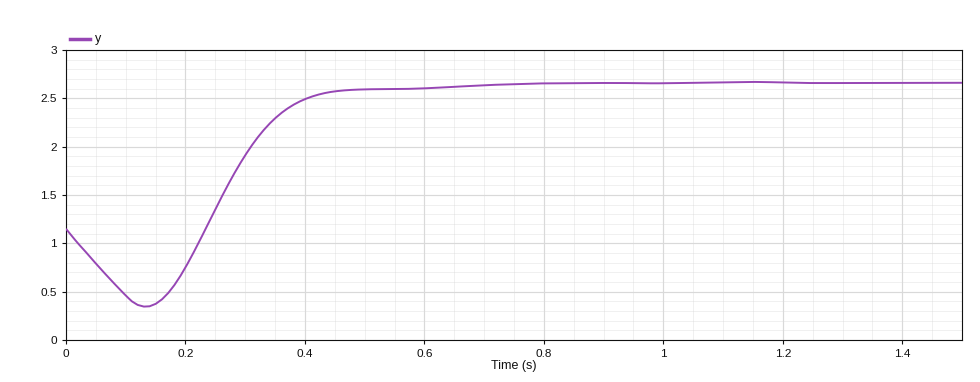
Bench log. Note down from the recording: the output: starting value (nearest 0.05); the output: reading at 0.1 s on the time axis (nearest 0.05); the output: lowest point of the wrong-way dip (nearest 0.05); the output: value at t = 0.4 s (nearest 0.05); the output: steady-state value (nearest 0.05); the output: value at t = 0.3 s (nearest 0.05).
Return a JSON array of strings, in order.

["1.15", "0.45", "0.35", "2.50", "2.65", "1.90"]
